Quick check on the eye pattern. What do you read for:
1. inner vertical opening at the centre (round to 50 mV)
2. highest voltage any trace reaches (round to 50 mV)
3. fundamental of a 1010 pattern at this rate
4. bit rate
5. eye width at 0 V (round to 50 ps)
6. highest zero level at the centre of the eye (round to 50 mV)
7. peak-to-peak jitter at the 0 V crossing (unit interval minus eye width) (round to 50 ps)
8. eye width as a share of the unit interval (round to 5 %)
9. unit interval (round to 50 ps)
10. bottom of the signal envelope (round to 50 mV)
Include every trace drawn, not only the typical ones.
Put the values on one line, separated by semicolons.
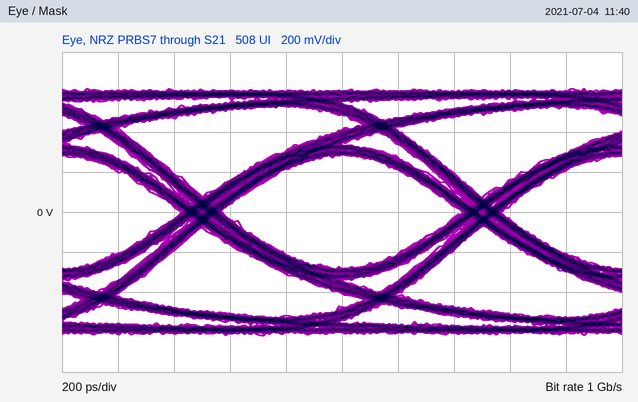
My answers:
550 mV; 600 mV; 500 MHz; 1 Gb/s; 850 ps; -300 mV; 150 ps; 85 %; 1.00 ns; -600 mV
